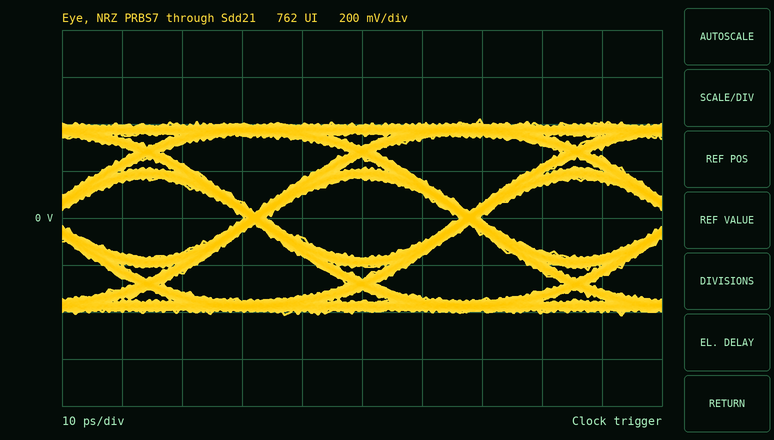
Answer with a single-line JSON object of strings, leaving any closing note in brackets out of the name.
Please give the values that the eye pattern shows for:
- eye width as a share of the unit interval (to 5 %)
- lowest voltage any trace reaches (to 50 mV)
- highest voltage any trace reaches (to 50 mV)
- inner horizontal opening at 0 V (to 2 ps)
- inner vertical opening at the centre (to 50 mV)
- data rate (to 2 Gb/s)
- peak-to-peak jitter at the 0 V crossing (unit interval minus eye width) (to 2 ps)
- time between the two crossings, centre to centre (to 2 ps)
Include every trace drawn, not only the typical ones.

{"eye width as a share of the unit interval": "90 %", "lowest voltage any trace reaches": "-400 mV", "highest voltage any trace reaches": "400 mV", "inner horizontal opening at 0 V": "32 ps", "inner vertical opening at the centre": "350 mV", "data rate": "28 Gb/s", "peak-to-peak jitter at the 0 V crossing (unit interval minus eye width)": "4 ps", "time between the two crossings, centre to centre": "36 ps"}
